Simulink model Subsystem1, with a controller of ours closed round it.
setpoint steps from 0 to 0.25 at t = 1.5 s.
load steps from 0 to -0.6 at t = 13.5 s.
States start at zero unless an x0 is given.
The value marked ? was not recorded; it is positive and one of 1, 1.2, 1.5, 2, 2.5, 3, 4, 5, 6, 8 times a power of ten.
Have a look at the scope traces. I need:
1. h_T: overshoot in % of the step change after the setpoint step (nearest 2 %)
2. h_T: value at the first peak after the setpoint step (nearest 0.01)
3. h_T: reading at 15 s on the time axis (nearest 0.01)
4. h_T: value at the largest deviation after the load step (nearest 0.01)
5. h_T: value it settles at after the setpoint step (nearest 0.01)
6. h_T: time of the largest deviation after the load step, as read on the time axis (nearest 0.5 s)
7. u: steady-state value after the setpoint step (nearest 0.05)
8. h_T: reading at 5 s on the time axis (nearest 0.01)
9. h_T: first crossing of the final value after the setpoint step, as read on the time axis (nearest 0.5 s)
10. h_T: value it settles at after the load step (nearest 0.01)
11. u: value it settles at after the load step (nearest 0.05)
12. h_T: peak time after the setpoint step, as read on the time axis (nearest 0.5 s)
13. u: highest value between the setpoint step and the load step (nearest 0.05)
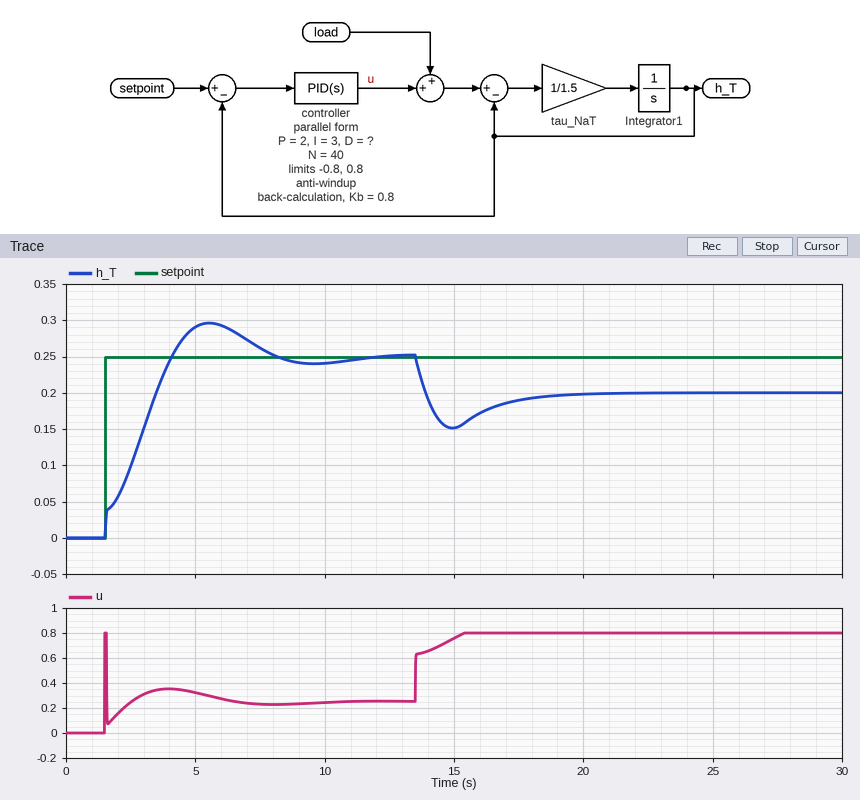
18 %
0.30
0.15
0.15
0.25
15.0 s
0.25
0.29
4.0 s
0.20
0.80
5.5 s
0.80
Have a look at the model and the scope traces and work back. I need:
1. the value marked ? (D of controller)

2.5
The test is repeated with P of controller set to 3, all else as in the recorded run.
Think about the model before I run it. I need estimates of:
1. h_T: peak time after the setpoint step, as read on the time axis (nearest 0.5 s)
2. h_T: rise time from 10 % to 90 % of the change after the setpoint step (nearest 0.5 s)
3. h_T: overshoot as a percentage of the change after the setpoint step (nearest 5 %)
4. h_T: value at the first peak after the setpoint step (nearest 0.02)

5.5 s
2.0 s
10 %
0.28
